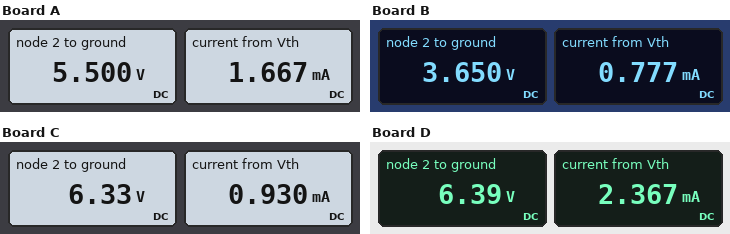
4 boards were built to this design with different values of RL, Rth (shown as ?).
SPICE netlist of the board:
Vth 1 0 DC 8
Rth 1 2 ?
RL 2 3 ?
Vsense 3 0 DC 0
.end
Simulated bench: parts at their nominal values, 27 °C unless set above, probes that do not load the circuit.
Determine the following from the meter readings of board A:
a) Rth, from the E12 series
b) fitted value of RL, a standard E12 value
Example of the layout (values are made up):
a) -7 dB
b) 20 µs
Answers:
a) 1.5 kΩ
b) 3.3 kΩ
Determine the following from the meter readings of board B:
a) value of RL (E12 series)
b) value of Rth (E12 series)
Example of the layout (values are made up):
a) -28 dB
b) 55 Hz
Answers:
a) 4.7 kΩ
b) 5.6 kΩ
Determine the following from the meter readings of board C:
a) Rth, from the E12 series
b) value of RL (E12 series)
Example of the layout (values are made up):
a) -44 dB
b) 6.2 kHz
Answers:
a) 1.8 kΩ
b) 6.8 kΩ
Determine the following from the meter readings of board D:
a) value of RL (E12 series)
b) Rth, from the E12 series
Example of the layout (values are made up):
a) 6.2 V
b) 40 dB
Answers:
a) 2.7 kΩ
b) 680 Ω
